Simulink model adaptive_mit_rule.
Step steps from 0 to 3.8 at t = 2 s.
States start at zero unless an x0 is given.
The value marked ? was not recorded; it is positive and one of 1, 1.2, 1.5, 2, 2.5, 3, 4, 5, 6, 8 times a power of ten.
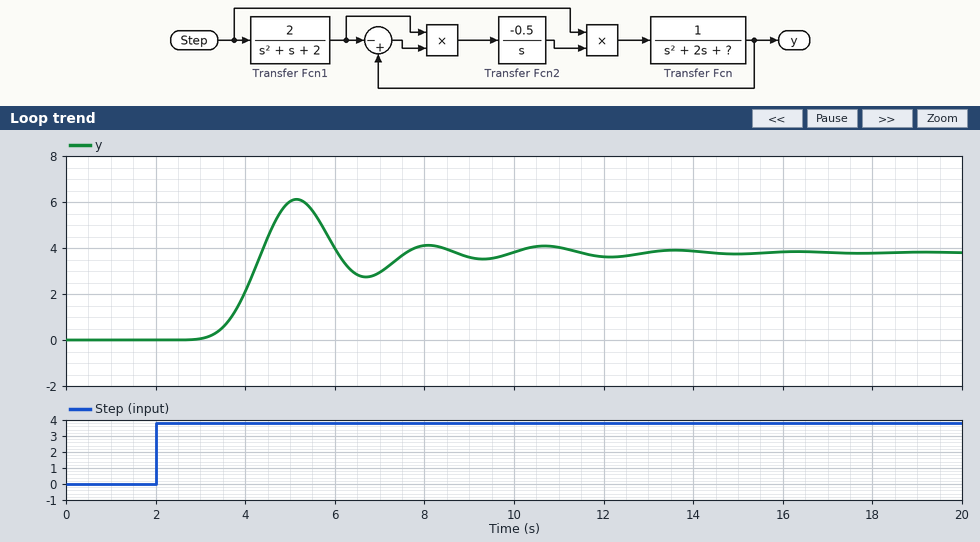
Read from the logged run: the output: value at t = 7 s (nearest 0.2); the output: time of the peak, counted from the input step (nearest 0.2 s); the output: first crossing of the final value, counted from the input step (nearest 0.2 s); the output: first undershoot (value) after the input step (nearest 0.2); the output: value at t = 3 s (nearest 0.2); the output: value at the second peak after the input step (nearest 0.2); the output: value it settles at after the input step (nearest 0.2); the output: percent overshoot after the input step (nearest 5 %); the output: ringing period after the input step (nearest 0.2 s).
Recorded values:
3.0
3.2 s
2.4 s
2.8
0.0
4.2
3.8
60 %
3.0 s
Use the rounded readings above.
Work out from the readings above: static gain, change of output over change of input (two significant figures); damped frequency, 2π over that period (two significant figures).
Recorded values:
1.0
2.1 rad/s
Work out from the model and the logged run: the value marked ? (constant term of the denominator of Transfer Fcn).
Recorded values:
6
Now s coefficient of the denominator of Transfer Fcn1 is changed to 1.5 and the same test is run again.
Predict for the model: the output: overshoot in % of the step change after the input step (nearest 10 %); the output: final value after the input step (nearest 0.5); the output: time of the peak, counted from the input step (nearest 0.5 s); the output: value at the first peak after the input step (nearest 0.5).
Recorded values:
30 %
4.0
3.5 s
5.0
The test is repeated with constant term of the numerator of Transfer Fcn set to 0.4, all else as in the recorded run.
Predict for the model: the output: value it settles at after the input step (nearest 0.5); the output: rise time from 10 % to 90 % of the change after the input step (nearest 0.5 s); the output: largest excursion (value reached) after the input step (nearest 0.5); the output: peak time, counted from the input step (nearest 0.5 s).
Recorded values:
4.0
1.5 s
4.0
4.0 s
